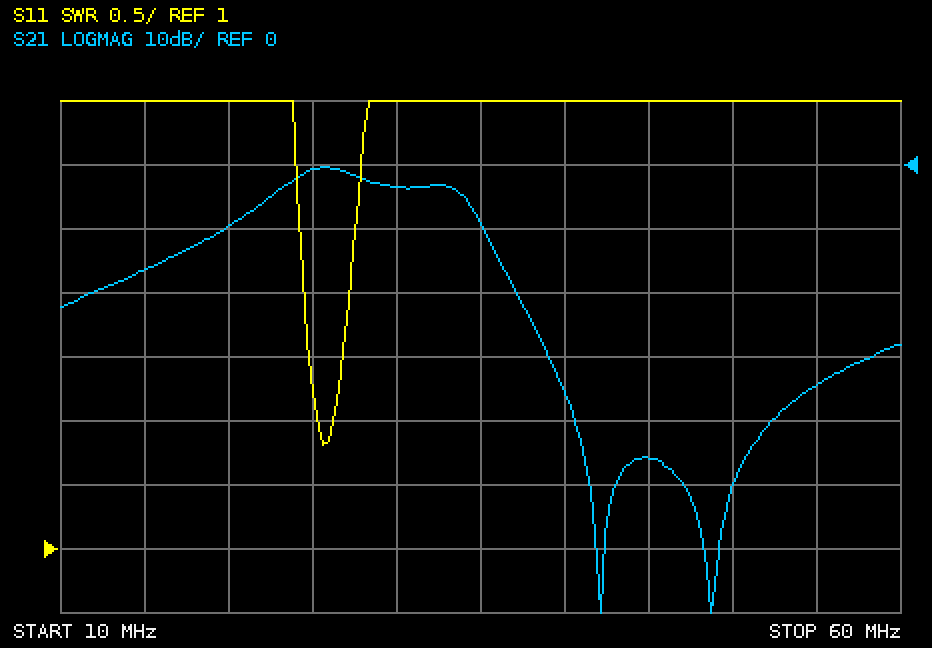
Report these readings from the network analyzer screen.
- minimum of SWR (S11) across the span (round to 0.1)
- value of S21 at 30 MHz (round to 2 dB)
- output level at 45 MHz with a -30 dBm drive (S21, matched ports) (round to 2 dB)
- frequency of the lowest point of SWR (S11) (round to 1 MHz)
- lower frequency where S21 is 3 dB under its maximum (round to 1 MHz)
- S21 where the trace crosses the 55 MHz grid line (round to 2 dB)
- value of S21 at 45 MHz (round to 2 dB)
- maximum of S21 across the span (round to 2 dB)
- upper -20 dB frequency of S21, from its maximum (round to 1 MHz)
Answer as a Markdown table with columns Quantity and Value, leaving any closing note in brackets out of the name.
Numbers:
| Quantity | Value |
|---|---|
| minimum of SWR (S11) across the span | 1.8 |
| value of S21 at 30 MHz | -4 dB |
| output level at 45 MHz with a -30 dBm drive (S21, matched ports) | -76 dBm |
| frequency of the lowest point of SWR (S11) | 26 MHz |
| lower frequency where S21 is 3 dB under its maximum | 23 MHz |
| S21 where the trace crosses the 55 MHz grid line | -34 dB |
| value of S21 at 45 MHz | -46 dB |
| maximum of S21 across the span | 0 dB |
| upper -20 dB frequency of S21, from its maximum | 37 MHz |
